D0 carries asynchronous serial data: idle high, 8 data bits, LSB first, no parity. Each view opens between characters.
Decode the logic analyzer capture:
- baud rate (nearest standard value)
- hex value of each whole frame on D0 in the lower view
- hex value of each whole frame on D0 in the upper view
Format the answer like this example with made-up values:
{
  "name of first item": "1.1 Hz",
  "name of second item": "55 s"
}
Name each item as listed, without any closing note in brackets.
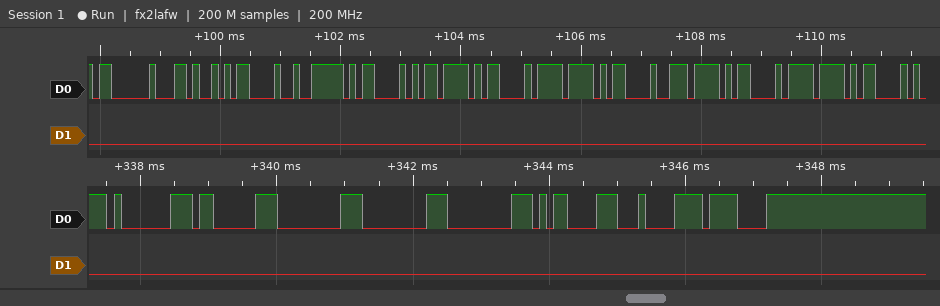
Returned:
{
  "baud rate": "9600 baud",
  "hex value of each whole frame on D0 in the lower view": "01, 03, 00, 00, 00, 0D, 84, 0F",
  "hex value of each whole frame on D0 in the upper view": "03, 2C, 0D, F2, 0D, ED, 0D, EF, 0D, EE, 0D, EF, 0D"
}
